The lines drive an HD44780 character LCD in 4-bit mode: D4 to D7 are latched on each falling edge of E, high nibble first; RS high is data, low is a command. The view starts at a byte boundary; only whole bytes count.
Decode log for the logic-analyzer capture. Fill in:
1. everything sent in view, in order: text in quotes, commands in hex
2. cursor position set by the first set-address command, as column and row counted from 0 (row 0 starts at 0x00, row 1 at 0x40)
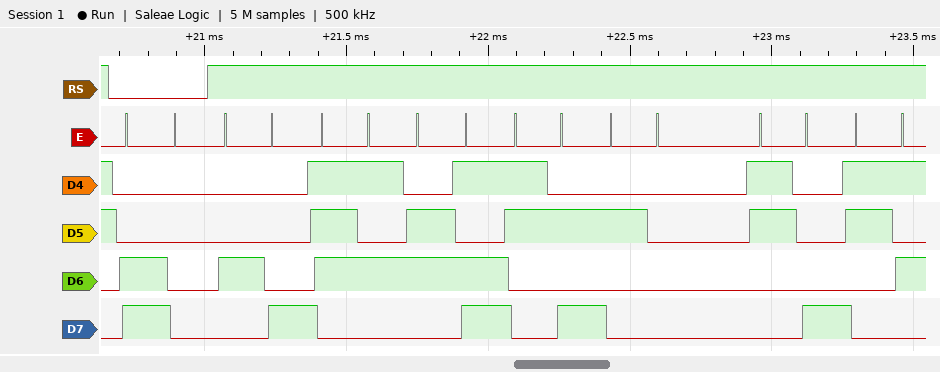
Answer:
0xC0 "Hum: 85"
column 0, row 1
